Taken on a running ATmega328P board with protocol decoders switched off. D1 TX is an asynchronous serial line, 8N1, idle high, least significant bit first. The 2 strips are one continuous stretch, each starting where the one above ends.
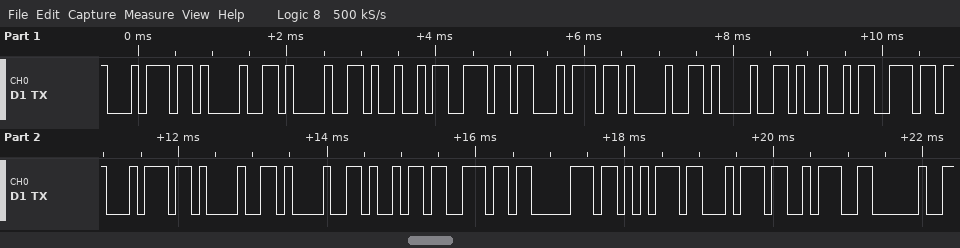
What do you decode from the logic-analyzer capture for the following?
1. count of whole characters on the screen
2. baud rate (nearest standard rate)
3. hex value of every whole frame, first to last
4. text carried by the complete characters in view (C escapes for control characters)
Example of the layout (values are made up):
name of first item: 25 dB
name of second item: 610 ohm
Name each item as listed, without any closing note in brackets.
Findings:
count of whole characters on the screen: 20
baud rate: 9600 baud
hex value of every whole frame, first to last: 74 21 21 49 6E 74 21 21 49 6E 74 21 21 69 6E 70 75 74 3A 20
text carried by the complete characters in view: "t!!Int!!Int!!input: "
